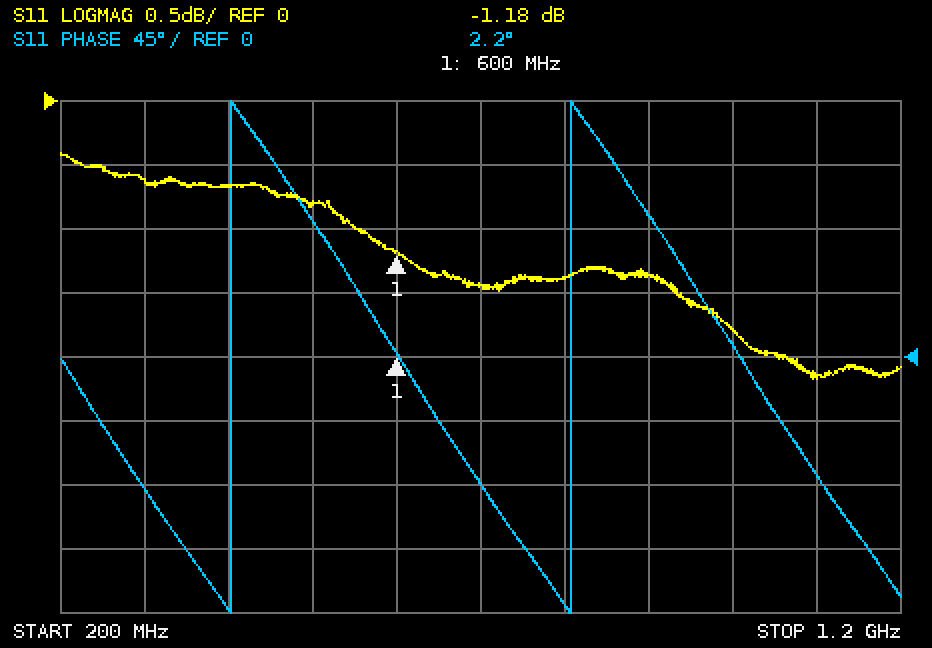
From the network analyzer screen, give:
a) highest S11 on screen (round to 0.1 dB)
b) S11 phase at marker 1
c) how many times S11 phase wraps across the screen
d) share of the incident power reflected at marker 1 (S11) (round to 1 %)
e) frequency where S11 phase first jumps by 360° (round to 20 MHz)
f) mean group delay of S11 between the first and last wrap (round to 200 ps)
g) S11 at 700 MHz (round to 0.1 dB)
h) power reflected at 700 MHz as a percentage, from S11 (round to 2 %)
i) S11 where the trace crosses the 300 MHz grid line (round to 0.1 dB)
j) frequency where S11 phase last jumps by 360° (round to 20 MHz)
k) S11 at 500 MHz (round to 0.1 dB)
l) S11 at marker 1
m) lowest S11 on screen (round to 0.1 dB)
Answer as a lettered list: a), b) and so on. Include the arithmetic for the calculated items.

a) -0.4 dB
b) 2.2°
c) 2
d) 10^(-1.18/10) ≈ 76 %
e) 400 MHz
f) 1 cycle / (800 MHz − 400 MHz) ≈ 2.50 ns, so 2.4 ns to the nearest 200 ps
g) -1.4 dB
h) 10^(-1.4/10) ≈ 72 %
i) -0.6 dB
j) 800 MHz
k) -0.8 dB
l) -1.18 dB
m) -2.2 dB
